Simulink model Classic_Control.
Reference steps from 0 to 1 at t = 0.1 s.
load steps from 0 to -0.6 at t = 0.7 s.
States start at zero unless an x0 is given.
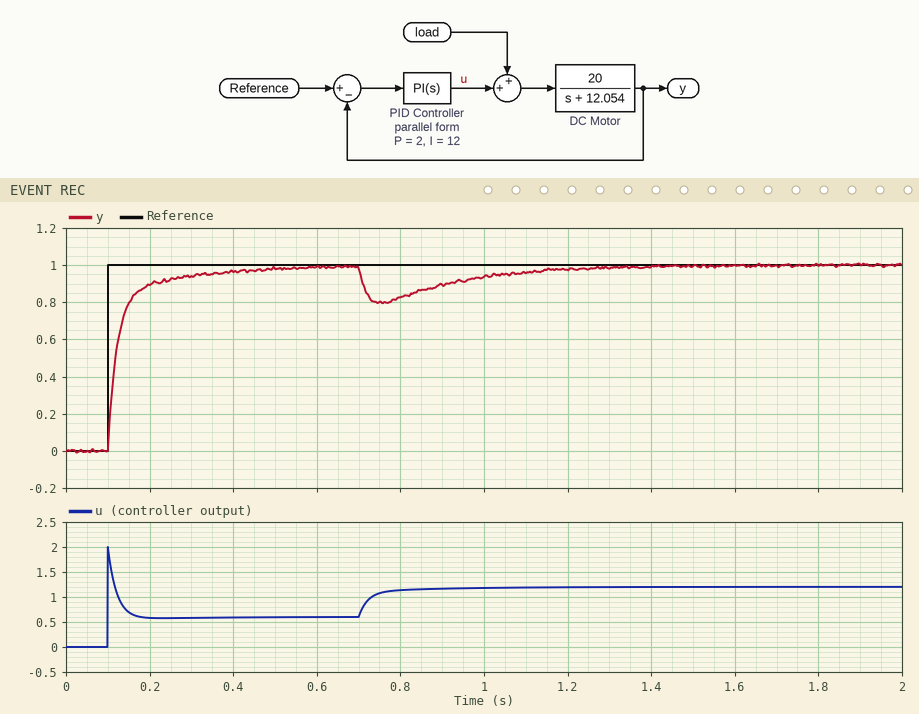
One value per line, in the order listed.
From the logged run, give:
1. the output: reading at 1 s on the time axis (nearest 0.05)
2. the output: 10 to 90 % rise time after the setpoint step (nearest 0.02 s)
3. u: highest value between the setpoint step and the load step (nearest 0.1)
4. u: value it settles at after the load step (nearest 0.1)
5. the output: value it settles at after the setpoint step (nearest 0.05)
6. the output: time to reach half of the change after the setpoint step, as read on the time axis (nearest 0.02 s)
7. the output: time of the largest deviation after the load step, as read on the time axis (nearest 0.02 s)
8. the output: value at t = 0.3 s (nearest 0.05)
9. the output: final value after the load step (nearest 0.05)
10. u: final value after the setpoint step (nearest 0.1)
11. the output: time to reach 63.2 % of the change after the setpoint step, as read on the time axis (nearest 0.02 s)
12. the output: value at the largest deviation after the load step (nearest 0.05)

0.95
0.10 s
2.0
1.2
1.00
0.12 s
0.76 s
0.95
1.00
0.6
0.12 s
0.80
